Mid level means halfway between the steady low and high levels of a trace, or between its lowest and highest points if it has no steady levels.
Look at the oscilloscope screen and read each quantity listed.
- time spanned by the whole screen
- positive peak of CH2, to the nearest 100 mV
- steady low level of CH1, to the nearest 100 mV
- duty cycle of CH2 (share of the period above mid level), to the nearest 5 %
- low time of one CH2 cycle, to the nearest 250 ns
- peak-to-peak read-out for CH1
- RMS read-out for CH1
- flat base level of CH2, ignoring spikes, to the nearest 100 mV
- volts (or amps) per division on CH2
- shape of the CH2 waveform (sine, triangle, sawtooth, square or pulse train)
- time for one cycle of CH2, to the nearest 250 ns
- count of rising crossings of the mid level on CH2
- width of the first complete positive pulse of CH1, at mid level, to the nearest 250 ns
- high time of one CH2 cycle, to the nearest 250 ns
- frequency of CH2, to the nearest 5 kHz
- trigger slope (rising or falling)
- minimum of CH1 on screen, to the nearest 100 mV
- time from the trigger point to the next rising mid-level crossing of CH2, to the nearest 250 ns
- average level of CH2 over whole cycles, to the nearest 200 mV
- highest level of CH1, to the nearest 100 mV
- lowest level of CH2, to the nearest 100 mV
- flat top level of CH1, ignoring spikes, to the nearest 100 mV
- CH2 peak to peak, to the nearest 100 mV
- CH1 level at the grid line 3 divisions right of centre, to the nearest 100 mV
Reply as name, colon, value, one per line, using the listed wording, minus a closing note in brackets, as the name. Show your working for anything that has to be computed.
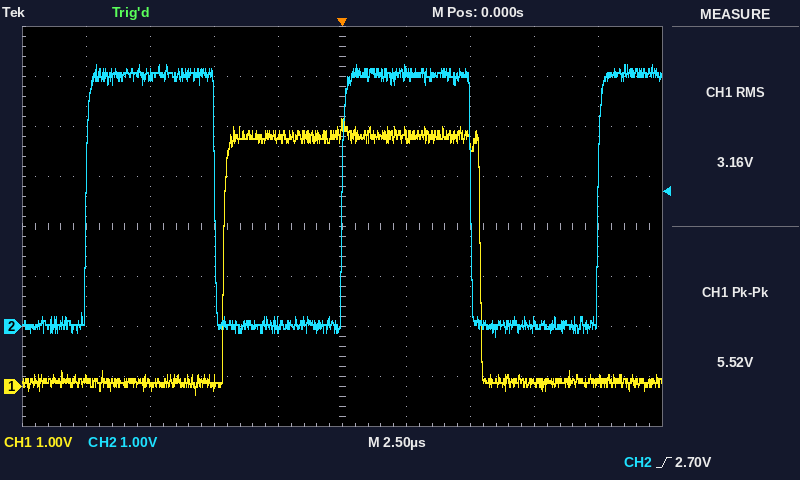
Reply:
time spanned by the whole screen: 25 µs
positive peak of CH2, to the nearest 100 mV: 5.2 V
steady low level of CH1, to the nearest 100 mV: 100 mV
duty cycle of CH2 (share of the period above mid level), to the nearest 5 %: 5.00 µs / 10.00 µs ≈ 50 %
low time of one CH2 cycle, to the nearest 250 ns: 5.00 µs
peak-to-peak read-out for CH1: 5.52 V
RMS read-out for CH1: 3.16 V
flat base level of CH2, ignoring spikes, to the nearest 100 mV: 0.0 V
volts (or amps) per division on CH2: 1 V
shape of the CH2 waveform: square
time for one cycle of CH2, to the nearest 250 ns: 10.00 µs
count of rising crossings of the mid level on CH2: 3
width of the first complete positive pulse of CH1, at mid level, to the nearest 250 ns: 10.00 µs
high time of one CH2 cycle, to the nearest 250 ns: 5.00 µs
frequency of CH2, to the nearest 5 kHz: 1 / 10.00 µs ≈ 100 kHz
trigger slope: rising
minimum of CH1 on screen, to the nearest 100 mV: -200 mV
time from the trigger point to the next rising mid-level crossing of CH2, to the nearest 250 ns: 10.00 µs
average level of CH2 over whole cycles, to the nearest 200 mV: 0.0 V + 0.5 × (5.2 V − (0.0 V)) ≈ 2.6 V
highest level of CH1, to the nearest 100 mV: 5.4 V
lowest level of CH2, to the nearest 100 mV: -200 mV
flat top level of CH1, ignoring spikes, to the nearest 100 mV: 5.0 V
CH2 peak to peak, to the nearest 100 mV: 5.2 V − (-200 mV) = 5.4 V
CH1 level at the grid line 3 divisions right of centre, to the nearest 100 mV: 100 mV
